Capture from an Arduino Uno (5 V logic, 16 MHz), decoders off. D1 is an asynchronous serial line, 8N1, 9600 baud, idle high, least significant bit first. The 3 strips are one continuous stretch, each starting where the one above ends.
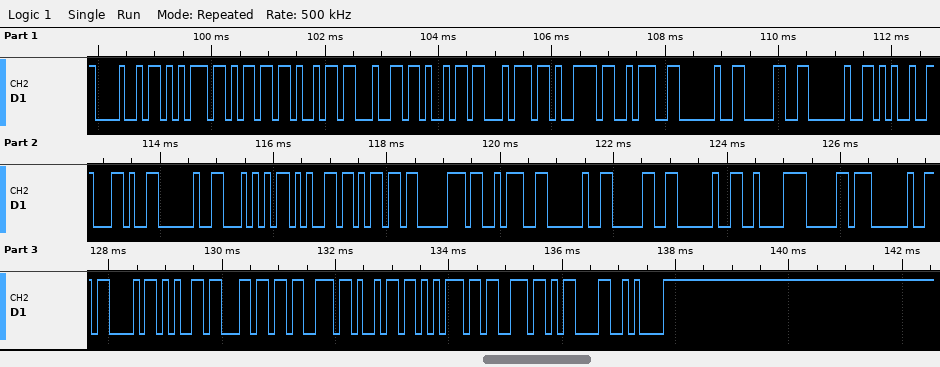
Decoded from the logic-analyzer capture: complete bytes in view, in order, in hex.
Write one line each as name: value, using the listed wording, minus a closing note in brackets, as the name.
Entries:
complete bytes in view, in order, in hex: 48 75 6D 69 64 69 74 79 3A 20 30 20 25 2C 20 54 65 6D 70 3A 20 30 20 C2 B0 20 43 65 6C 73 69 75 73 0D 0A
